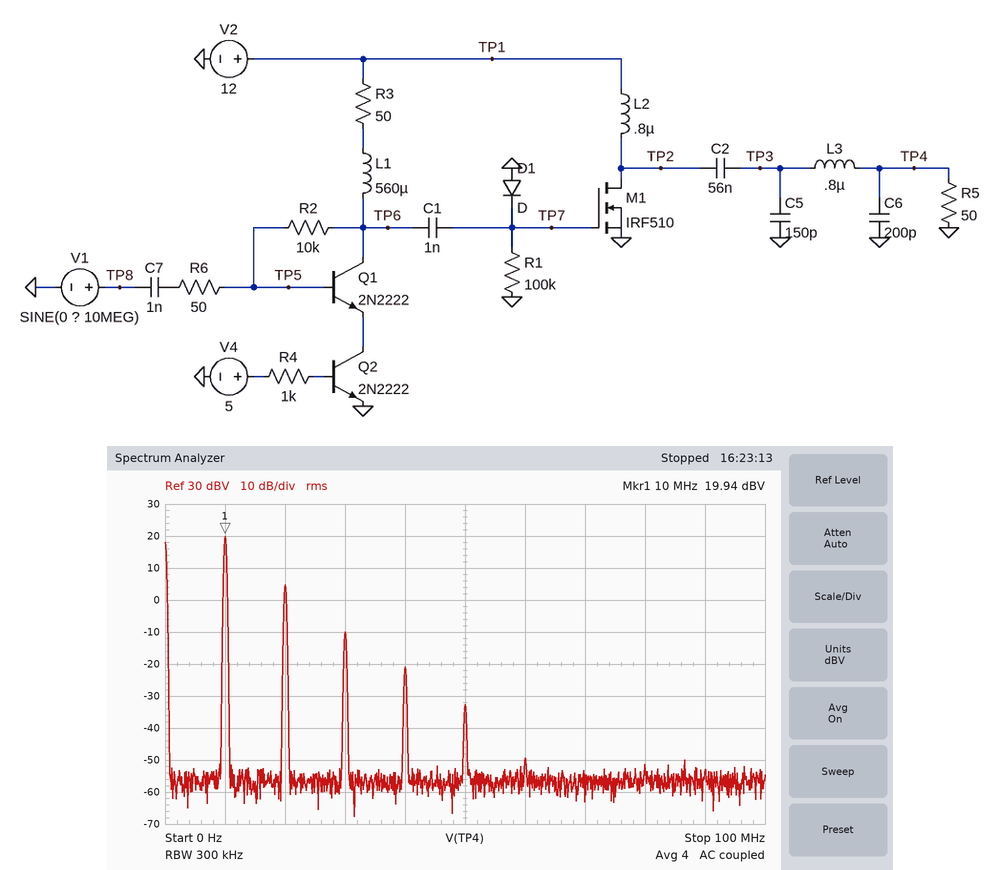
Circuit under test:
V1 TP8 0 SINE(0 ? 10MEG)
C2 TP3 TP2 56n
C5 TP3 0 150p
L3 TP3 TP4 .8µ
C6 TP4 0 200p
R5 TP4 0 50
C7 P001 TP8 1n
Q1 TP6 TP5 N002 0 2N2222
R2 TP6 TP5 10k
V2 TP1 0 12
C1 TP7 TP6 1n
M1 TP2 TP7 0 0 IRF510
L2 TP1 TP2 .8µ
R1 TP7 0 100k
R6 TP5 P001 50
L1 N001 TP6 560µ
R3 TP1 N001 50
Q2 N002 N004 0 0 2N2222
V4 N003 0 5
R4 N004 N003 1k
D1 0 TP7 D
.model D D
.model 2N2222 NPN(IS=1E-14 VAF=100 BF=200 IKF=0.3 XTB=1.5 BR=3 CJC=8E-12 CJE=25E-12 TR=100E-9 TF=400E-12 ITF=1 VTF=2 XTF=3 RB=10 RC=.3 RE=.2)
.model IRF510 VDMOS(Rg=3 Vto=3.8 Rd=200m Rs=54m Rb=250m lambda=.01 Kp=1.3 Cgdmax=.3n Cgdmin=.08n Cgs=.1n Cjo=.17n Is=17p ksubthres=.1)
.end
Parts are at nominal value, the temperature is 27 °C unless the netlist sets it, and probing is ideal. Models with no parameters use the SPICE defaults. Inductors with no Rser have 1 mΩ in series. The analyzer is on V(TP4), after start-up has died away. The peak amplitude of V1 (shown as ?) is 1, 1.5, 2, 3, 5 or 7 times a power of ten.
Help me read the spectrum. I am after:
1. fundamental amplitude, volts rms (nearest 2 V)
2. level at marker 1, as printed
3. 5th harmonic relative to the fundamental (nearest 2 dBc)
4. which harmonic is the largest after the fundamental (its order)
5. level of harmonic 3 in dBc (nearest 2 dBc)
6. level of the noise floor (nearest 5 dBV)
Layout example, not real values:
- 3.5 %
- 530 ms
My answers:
- 10 V
- 19.94 dBV
- -52 dBc
- 2
- -30 dBc
- -55 dBV
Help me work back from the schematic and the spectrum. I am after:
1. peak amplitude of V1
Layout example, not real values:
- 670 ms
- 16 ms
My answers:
- 2 V
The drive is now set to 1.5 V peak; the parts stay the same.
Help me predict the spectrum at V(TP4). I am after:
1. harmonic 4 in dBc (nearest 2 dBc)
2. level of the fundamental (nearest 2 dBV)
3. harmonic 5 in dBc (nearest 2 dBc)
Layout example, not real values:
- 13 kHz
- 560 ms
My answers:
- -42 dBc
- 20 dBV
- -56 dBc
